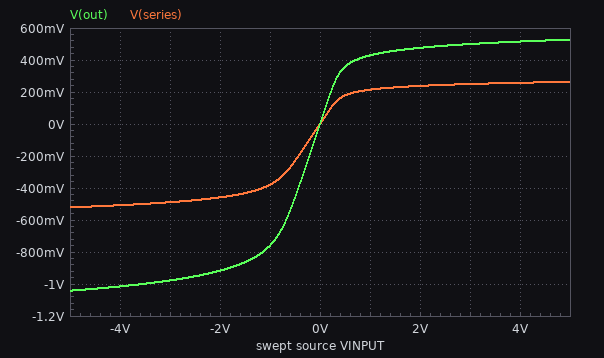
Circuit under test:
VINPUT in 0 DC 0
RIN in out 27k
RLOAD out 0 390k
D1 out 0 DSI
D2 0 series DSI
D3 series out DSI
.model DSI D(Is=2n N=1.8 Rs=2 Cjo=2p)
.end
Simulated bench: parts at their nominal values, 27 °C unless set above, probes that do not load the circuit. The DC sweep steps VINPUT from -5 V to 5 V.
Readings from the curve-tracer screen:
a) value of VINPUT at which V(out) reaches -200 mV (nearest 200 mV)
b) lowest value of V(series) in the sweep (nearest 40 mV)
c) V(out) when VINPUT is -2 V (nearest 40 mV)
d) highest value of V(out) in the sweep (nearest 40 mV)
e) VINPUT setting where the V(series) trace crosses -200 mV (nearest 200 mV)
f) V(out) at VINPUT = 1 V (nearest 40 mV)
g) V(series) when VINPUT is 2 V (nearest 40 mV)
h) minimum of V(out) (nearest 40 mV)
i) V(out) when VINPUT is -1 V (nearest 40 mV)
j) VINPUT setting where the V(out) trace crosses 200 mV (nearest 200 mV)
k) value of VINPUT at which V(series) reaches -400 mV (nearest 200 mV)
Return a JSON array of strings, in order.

["-200 mV", "-520 mV", "-920 mV", "520 mV", "-400 mV", "440 mV", "240 mV", "-1.04 V", "-760 mV", "200 mV", "-1.2 V"]
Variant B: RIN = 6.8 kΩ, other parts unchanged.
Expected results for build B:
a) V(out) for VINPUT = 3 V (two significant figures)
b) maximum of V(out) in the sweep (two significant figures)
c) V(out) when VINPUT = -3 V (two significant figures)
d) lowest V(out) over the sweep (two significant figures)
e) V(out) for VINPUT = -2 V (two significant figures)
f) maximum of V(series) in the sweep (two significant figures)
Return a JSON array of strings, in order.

["560 mV", "590 mV", "-1.1 V", "-1.2 V", "-1.0 V", "300 mV"]
